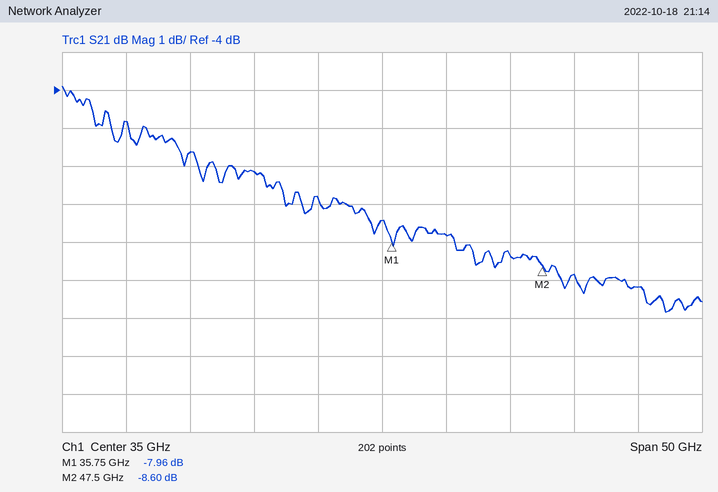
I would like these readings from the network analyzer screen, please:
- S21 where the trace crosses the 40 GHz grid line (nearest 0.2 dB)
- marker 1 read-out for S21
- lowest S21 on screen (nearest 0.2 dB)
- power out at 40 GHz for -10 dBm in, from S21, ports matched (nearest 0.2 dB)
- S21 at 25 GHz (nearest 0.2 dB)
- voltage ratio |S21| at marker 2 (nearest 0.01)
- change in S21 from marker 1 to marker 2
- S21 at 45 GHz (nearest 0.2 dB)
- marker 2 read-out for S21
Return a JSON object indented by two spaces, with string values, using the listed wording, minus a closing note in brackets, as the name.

{
  "S21 where the trace crosses the 40 GHz grid line": "-7.8 dB",
  "marker 1 read-out for S21": "-7.96 dB",
  "lowest S21 on screen": "-9.8 dB",
  "power out at 40 GHz for -10 dBm in, from S21, ports matched": "-17.8 dBm",
  "S21 at 25 GHz": "-6.2 dB",
  "voltage ratio |S21| at marker 2": "0.37",
  "change in S21 from marker 1 to marker 2": "-0.64 dB",
  "S21 at 45 GHz": "-8.4 dB",
  "marker 2 read-out for S21": "-8.60 dB"
}
